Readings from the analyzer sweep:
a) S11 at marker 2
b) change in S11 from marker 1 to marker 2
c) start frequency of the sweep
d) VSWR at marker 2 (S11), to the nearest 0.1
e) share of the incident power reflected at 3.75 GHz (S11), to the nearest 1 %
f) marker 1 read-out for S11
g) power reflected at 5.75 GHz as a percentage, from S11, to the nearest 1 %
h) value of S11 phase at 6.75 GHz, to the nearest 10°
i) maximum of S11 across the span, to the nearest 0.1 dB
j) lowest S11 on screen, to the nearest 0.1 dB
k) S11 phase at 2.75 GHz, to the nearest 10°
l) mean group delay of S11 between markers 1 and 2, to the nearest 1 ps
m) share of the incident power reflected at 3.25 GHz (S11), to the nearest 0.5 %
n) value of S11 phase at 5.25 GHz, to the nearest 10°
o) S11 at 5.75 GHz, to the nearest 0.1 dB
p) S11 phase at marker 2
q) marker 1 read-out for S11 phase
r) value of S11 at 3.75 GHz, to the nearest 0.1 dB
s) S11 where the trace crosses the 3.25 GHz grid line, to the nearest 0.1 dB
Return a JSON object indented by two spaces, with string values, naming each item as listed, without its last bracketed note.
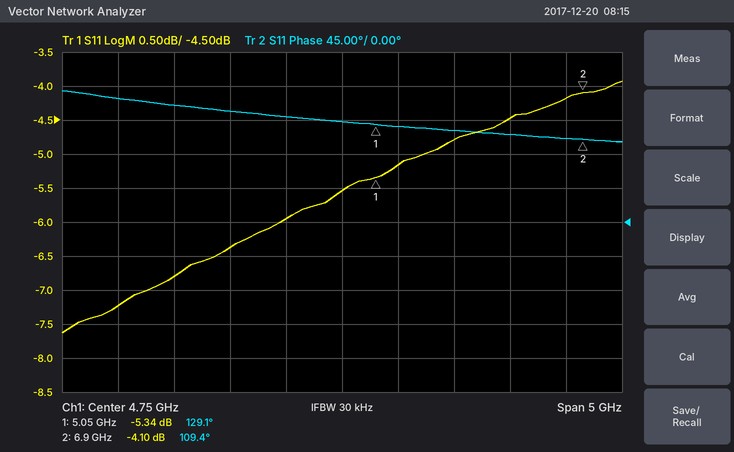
{
  "S11 at marker 2": "-4.10 dB",
  "change in S11 from marker 1 to marker 2": "1.24 dB",
  "start frequency of the sweep": "2.25 GHz",
  "VSWR at marker 2 (S11), to the nearest 0.1": "4.3",
  "share of the incident power reflected at 3.75 GHz (S11), to the nearest 1 %": "23 %",
  "marker 1 read-out for S11": "-5.34 dB",
  "power reflected at 5.75 GHz as a percentage, from S11, to the nearest 1 %": "33 %",
  "value of S11 phase at 6.75 GHz, to the nearest 10°": "110°",
  "maximum of S11 across the span, to the nearest 0.1 dB": "-3.9 dB",
  "lowest S11 on screen, to the nearest 0.1 dB": "-7.6 dB",
  "S11 phase at 2.75 GHz, to the nearest 10°": "160°",
  "mean group delay of S11 between markers 1 and 2, to the nearest 1 ps": "30 ps",
  "share of the incident power reflected at 3.25 GHz (S11), to the nearest 0.5 %": "21.0 %",
  "value of S11 phase at 5.25 GHz, to the nearest 10°": "130°",
  "S11 at 5.75 GHz, to the nearest 0.1 dB": "-4.8 dB",
  "S11 phase at marker 2": "109.4°",
  "marker 1 read-out for S11 phase": "129.1°",
  "value of S11 at 3.75 GHz, to the nearest 0.1 dB": "-6.4 dB",
  "S11 where the trace crosses the 3.25 GHz grid line, to the nearest 0.1 dB": "-6.8 dB"
}
